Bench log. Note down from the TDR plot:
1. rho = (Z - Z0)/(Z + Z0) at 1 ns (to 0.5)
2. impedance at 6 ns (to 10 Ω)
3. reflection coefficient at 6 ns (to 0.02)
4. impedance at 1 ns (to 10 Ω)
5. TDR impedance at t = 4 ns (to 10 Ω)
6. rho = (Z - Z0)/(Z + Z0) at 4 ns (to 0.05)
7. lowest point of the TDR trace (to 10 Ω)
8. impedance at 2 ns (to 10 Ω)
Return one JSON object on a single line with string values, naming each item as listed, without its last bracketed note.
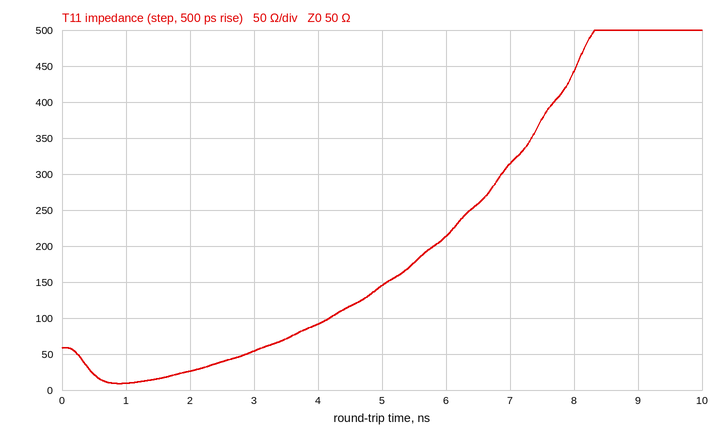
{"rho = (Z - Z0)/(Z + Z0) at 1 ns": "-0.5", "impedance at 6 ns": "210 Ω", "reflection coefficient at 6 ns": "+0.62", "impedance at 1 ns": "10 Ω", "TDR impedance at t = 4 ns": "90 Ω", "rho = (Z - Z0)/(Z + Z0) at 4 ns": "+0.30", "lowest point of the TDR trace": "10 Ω", "impedance at 2 ns": "30 Ω"}
